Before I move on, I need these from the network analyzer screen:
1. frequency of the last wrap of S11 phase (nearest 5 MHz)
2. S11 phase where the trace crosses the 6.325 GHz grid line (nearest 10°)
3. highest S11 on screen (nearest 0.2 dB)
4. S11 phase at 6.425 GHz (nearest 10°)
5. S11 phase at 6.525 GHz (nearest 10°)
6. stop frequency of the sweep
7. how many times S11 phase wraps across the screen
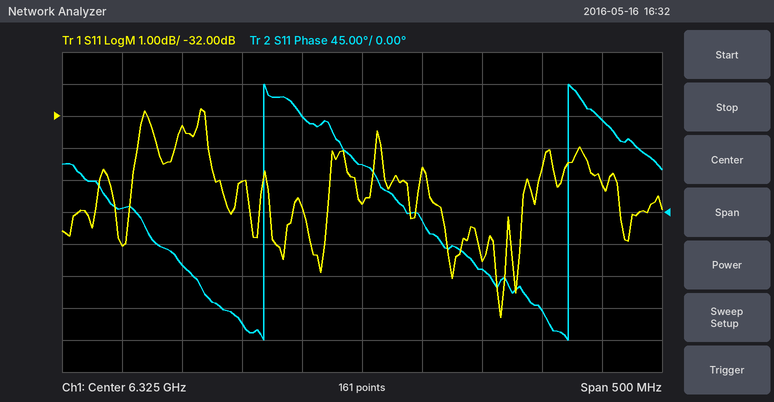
6.495 GHz
70°
-31.8 dB
-80°
130°
6.575 GHz
2
